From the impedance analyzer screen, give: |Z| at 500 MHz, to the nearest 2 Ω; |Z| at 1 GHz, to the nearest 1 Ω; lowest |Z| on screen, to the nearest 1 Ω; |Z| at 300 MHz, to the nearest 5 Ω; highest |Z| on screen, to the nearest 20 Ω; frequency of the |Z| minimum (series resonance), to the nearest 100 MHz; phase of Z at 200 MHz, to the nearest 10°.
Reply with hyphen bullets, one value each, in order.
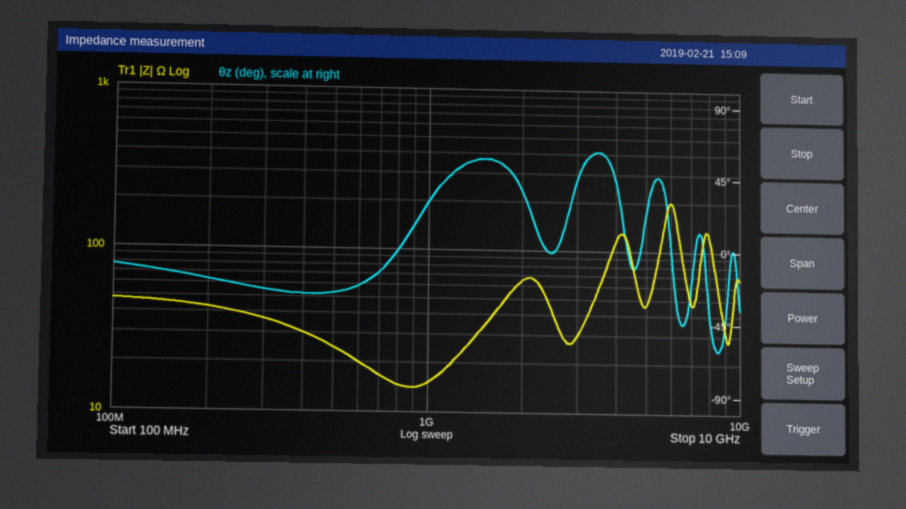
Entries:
- 24 Ω
- 15 Ω
- 14 Ω
- 35 Ω
- 200 Ω
- 900 MHz
- -20°
